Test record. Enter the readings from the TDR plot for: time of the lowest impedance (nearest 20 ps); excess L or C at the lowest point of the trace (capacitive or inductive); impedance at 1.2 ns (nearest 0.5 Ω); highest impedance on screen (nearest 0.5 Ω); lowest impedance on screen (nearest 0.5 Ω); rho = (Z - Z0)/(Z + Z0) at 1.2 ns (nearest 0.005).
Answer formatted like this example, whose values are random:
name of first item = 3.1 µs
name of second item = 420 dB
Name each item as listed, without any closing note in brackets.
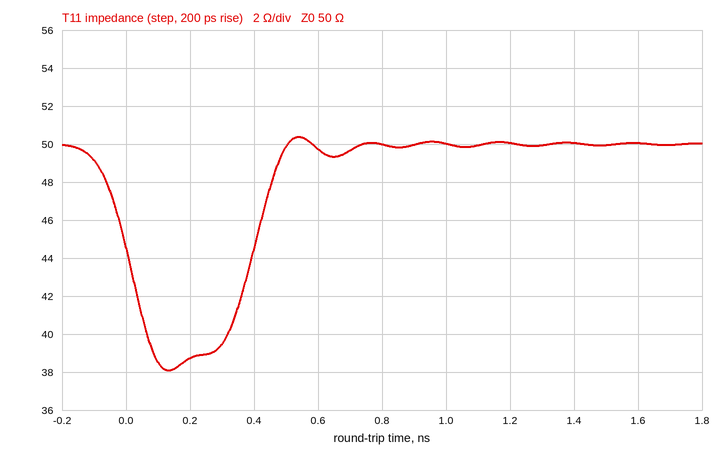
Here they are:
time of the lowest impedance = 140 ps
excess L or C at the lowest point of the trace = capacitive
impedance at 1.2 ns = 50.0 Ω
highest impedance on screen = 50.5 Ω
lowest impedance on screen = 38.0 Ω
rho = (Z - Z0)/(Z + Z0) at 1.2 ns = 0.000
